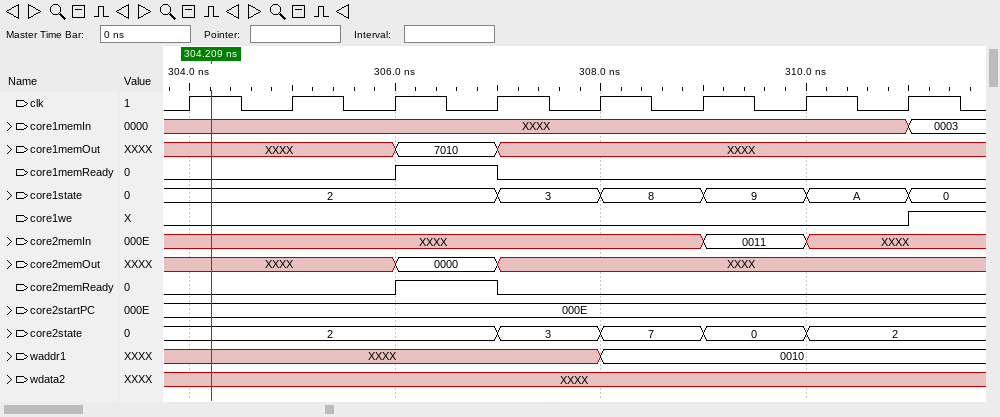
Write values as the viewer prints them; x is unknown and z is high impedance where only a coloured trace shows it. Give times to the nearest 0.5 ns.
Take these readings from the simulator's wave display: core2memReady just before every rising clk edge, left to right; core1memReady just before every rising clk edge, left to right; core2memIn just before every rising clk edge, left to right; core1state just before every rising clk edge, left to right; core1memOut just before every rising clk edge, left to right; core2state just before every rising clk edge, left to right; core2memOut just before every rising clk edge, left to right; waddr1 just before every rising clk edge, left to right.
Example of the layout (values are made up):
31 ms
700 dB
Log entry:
0 0 0 1 0 0 0 0
0 0 0 1 0 0 0 0
XXXX, XXXX, XXXX, XXXX, XXXX, XXXX, 0011, XXXX
2, 2, 2, 2, 3, 8, 9, A
XXXX, XXXX, XXXX, 7010, XXXX, XXXX, XXXX, XXXX
2, 2, 2, 2, 3, 7, 0, 2
XXXX, XXXX, XXXX, 0000, XXXX, XXXX, XXXX, XXXX
XXXX, XXXX, XXXX, XXXX, XXXX, 0010, 0010, 0010
